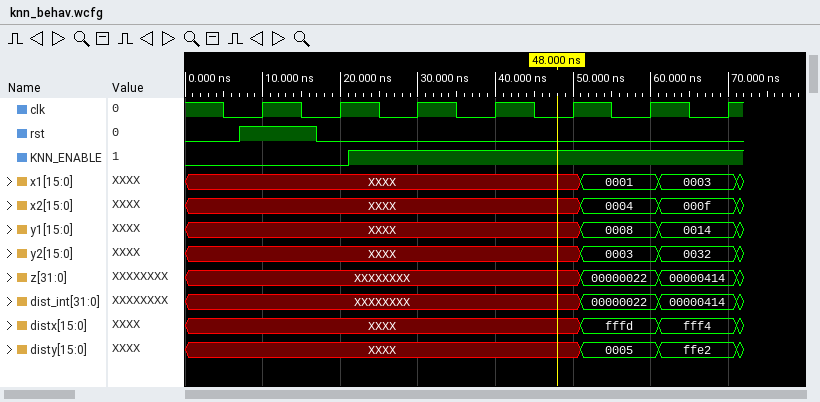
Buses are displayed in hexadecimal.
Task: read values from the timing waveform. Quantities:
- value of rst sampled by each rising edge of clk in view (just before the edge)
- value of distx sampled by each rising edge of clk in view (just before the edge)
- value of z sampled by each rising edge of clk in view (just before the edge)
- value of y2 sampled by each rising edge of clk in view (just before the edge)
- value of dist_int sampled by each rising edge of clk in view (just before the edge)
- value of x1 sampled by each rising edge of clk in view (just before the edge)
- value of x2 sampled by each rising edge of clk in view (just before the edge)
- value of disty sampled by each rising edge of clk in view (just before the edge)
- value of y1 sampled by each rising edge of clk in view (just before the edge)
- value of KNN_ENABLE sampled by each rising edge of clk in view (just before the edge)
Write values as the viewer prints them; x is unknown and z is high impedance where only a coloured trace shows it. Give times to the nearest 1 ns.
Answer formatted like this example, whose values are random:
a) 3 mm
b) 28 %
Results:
a) 1 0 0 0 0 0 0
b) XXXX, XXXX, XXXX, XXXX, XXXX, fffd, fff4
c) XXXXXXXX, XXXXXXXX, XXXXXXXX, XXXXXXXX, XXXXXXXX, 00000022, 00000414
d) XXXX, XXXX, XXXX, XXXX, XXXX, 0003, 0032
e) XXXXXXXX, XXXXXXXX, XXXXXXXX, XXXXXXXX, XXXXXXXX, 00000022, 00000414
f) XXXX, XXXX, XXXX, XXXX, XXXX, 0001, 0003
g) XXXX, XXXX, XXXX, XXXX, XXXX, 0004, 000f
h) XXXX, XXXX, XXXX, XXXX, XXXX, 0005, ffe2
i) XXXX, XXXX, XXXX, XXXX, XXXX, 0008, 0014
j) 0 0 1 1 1 1 1
